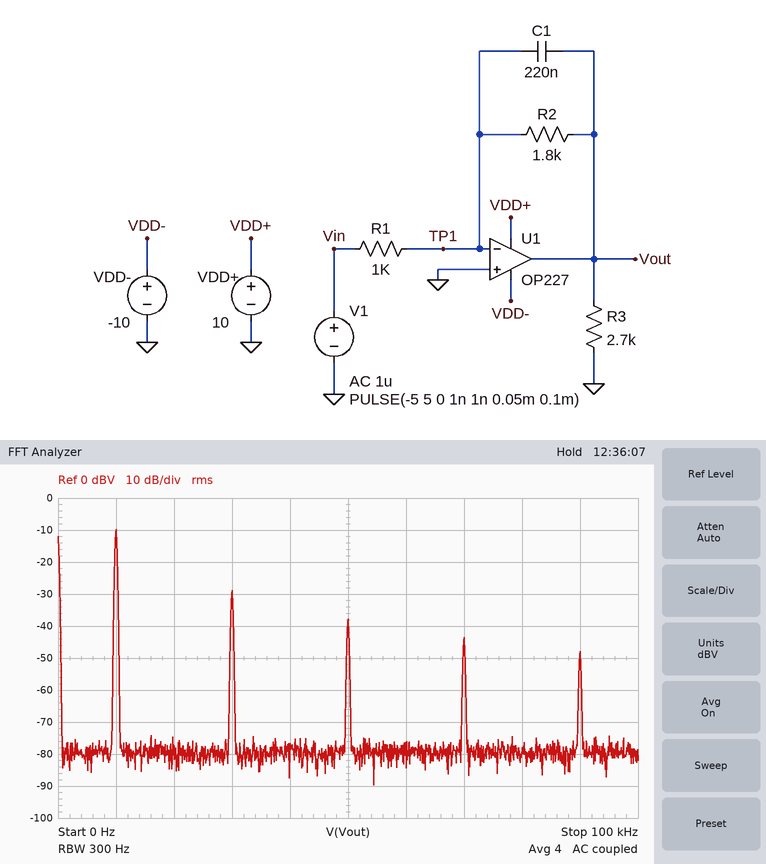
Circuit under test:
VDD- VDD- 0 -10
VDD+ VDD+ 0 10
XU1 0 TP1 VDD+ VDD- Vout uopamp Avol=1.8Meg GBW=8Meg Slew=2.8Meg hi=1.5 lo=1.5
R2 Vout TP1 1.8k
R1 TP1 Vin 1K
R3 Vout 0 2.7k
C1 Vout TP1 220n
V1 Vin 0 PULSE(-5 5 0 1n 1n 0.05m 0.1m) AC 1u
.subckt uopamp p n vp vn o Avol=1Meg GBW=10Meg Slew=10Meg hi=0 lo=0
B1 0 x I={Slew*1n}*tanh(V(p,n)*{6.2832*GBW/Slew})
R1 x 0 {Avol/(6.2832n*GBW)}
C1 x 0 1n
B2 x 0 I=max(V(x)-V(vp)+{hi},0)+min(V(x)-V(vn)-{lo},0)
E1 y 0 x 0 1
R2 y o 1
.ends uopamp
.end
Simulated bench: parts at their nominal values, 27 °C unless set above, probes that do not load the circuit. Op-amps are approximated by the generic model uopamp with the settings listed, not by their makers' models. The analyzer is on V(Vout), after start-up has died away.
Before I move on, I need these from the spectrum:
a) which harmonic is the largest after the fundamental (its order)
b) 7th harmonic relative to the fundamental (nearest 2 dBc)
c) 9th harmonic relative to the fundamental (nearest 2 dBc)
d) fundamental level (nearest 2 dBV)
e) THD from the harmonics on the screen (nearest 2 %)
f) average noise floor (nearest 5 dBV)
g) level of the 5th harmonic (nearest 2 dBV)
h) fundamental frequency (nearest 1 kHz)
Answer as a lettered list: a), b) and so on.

a) 3
b) -34 dBc
c) -38 dBc
d) -10 dBV
e) 12 %
f) -80 dBV
g) -38 dBV
h) 10 kHz
